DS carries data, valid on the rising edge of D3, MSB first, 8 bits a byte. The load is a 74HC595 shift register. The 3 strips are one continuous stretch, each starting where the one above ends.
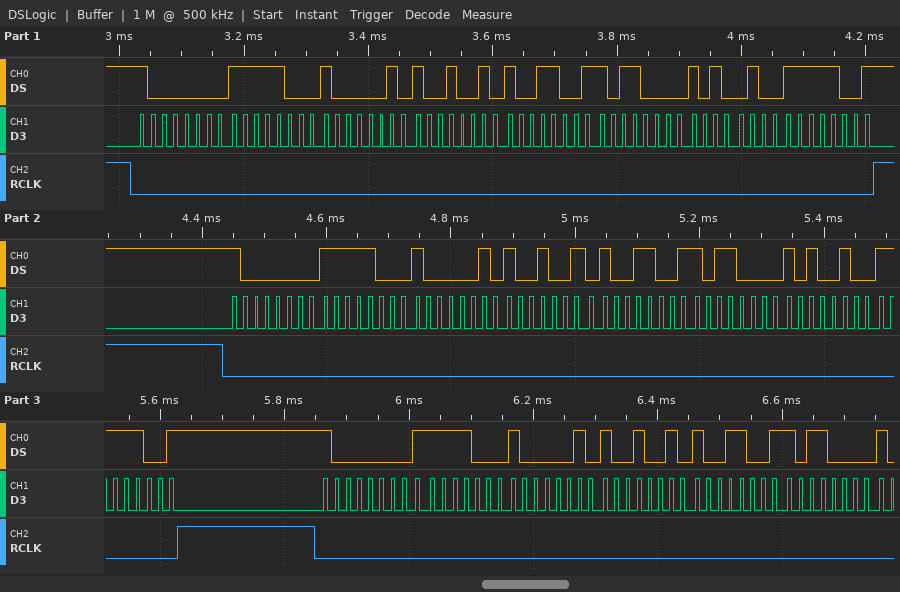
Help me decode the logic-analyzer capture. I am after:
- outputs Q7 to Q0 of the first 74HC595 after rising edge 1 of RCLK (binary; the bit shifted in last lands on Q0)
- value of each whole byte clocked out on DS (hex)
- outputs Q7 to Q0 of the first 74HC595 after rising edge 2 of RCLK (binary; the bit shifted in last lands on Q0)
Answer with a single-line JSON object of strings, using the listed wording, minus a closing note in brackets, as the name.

{"outputs Q7 to Q0 of the first 74HC595 after rising edge 1 of RCLK": "11111001", "value of each whole byte clocked out on DS": "0x80 0xF8 0x82 0x92 0x99 0xB0 0xA4 0xF9 0x80 0xF8 0x82 0x92 0x99 0xB0 0xA4 0xF9 0x80 0xF8 0x82 0x92 0x99 0xB0", "outputs Q7 to Q0 of the first 74HC595 after rising edge 2 of RCLK": "11111001"}
